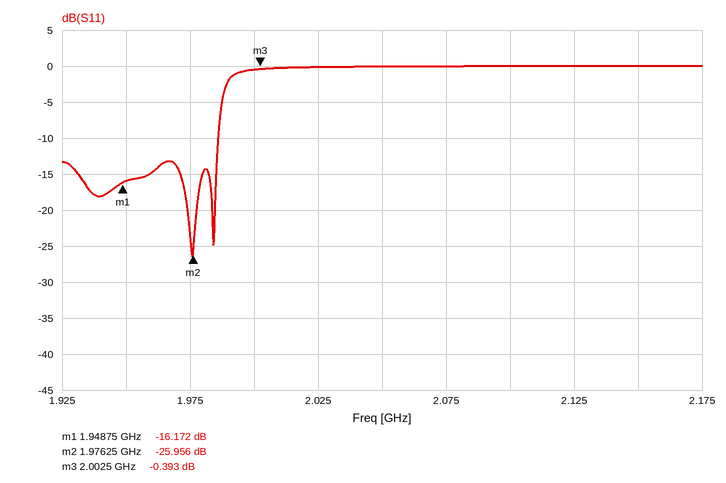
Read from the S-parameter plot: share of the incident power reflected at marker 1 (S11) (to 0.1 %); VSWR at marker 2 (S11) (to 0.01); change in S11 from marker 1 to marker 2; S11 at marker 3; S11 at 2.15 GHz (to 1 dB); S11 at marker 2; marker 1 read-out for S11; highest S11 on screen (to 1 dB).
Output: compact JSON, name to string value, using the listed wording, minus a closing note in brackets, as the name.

{"share of the incident power reflected at marker 1 (S11)": "2.4 %", "VSWR at marker 2 (S11)": "1.11", "change in S11 from marker 1 to marker 2": "-9.784 dB", "S11 at marker 3": "-0.393 dB", "S11 at 2.15 GHz": "0 dB", "S11 at marker 2": "-25.956 dB", "marker 1 read-out for S11": "-16.172 dB", "highest S11 on screen": "0 dB"}
